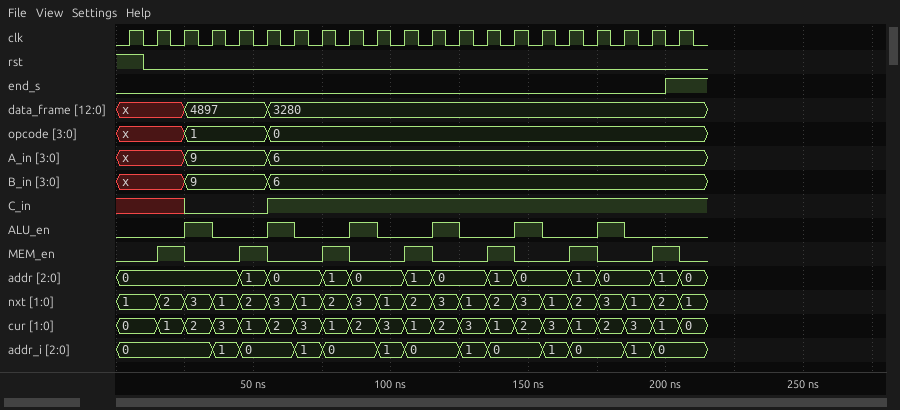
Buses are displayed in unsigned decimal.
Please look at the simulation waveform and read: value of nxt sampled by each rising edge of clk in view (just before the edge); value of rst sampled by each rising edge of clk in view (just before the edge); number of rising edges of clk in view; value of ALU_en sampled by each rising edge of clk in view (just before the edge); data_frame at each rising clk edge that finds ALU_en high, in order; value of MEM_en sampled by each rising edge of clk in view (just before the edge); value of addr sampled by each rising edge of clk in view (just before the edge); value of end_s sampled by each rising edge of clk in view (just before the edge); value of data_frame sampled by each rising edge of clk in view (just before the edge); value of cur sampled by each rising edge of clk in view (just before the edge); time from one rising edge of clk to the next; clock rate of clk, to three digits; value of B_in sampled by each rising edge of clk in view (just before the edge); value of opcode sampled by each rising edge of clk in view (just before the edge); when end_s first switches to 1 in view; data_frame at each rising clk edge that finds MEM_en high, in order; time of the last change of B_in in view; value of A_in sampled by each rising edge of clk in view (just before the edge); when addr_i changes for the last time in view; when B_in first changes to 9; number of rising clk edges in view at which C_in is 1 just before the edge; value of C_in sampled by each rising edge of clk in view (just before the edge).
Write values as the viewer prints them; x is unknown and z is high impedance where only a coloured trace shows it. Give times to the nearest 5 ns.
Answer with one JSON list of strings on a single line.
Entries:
["1, 1, 2, 3, 1, 2, 3, 1, 2, 3, 1, 2, 3, 1, 2, 3, 1, 2, 3, 1, 2", "1 0 0 0 0 0 0 0 0 0 0 0 0 0 0 0 0 0 0 0 0", "21", "0 0 0 1 0 0 1 0 0 1 0 0 1 0 0 1 0 0 1 0 0", "4897, 3280, 3280, 3280, 3280, 3280", "0 0 1 0 0 1 0 0 1 0 0 1 0 0 1 0 0 1 0 0 1", "0, 0, 0, 0, 0, 1, 0, 0, 1, 0, 0, 1, 0, 0, 1, 0, 0, 1, 0, 0, 1", "0 0 0 0 0 0 0 0 0 0 0 0 0 0 0 0 0 0 0 0 1", "x, x, x, 4897, 4897, 4897, 3280, 3280, 3280, 3280, 3280, 3280, 3280, 3280, 3280, 3280, 3280, 3280, 3280, 3280, 3280", "0, 0, 1, 2, 3, 1, 2, 3, 1, 2, 3, 1, 2, 3, 1, 2, 3, 1, 2, 3, 1", "10 ns", "100 MHz", "x, x, x, 9, 9, 9, 6, 6, 6, 6, 6, 6, 6, 6, 6, 6, 6, 6, 6, 6, 6", "x, x, x, 1, 1, 1, 0, 0, 0, 0, 0, 0, 0, 0, 0, 0, 0, 0, 0, 0, 0", "200 ns", "x, 4897, 3280, 3280, 3280, 3280, 3280", "55 ns", "x, x, x, 9, 9, 9, 6, 6, 6, 6, 6, 6, 6, 6, 6, 6, 6, 6, 6, 6, 6", "195 ns", "25 ns", "15", "x x x 0 0 0 1 1 1 1 1 1 1 1 1 1 1 1 1 1 1"]
